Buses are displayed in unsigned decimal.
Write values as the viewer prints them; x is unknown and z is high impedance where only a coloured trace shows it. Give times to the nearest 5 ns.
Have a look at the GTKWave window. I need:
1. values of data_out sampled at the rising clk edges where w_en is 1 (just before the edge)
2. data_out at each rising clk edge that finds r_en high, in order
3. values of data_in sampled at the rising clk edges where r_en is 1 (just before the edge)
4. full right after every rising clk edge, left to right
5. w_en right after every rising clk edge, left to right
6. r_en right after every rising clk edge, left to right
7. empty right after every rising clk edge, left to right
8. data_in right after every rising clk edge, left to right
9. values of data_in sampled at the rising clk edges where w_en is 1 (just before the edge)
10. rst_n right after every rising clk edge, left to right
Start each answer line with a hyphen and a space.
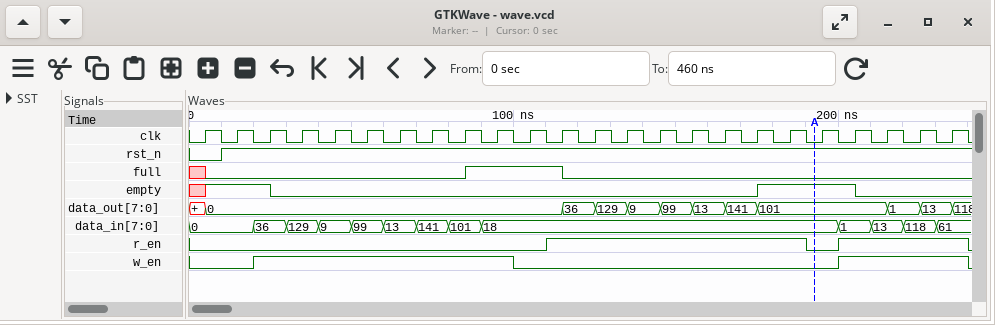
- 0, 0, 0, 0, 0, 0, 0, 0, 101, 101, 1, 13
- 0, 36, 129, 9, 99, 13, 141, 101, 101, 101, 1, 13
- 18, 18, 18, 18, 18, 18, 18, 18, 1, 13, 118, 61
- 0 0 0 0 0 0 0 0 1 1 1 0 0 0 0 0 0 0 0 0 0 0 0 0
- 0 0 1 1 1 1 1 1 1 1 0 0 0 0 0 0 0 0 0 0 1 1 1 1
- 0 0 0 0 0 0 0 0 0 0 0 1 1 1 1 1 1 1 1 0 1 1 1 1
- 1 1 0 0 0 0 0 0 0 0 0 0 0 0 0 0 0 1 1 1 0 0 0 0
- 0, 0, 36, 129, 9, 99, 13, 141, 101, 18, 18, 18, 18, 18, 18, 18, 18, 18, 18, 18, 1, 13, 118, 61
- 36, 129, 9, 99, 13, 141, 101, 18, 1, 13, 118, 61
- 0 1 1 1 1 1 1 1 1 1 1 1 1 1 1 1 1 1 1 1 1 1 1 1
